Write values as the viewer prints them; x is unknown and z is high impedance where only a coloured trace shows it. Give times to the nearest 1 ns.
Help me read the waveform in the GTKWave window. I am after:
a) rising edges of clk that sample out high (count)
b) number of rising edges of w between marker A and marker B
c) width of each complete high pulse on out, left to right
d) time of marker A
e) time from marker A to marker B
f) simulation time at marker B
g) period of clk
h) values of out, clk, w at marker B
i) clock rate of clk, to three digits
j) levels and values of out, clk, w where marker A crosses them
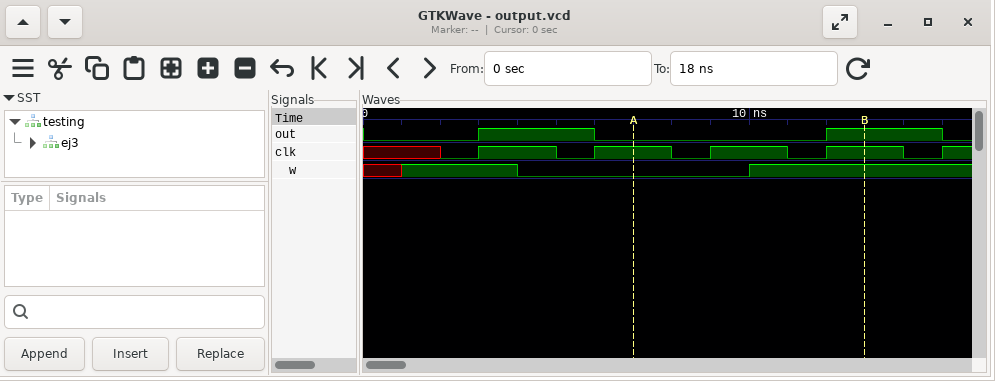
2
1
3 ns, 3 ns
7 ns
6 ns
13 ns
3 ns
out=1, clk=1, w=1
333 MHz
out=0, clk=1, w=0
